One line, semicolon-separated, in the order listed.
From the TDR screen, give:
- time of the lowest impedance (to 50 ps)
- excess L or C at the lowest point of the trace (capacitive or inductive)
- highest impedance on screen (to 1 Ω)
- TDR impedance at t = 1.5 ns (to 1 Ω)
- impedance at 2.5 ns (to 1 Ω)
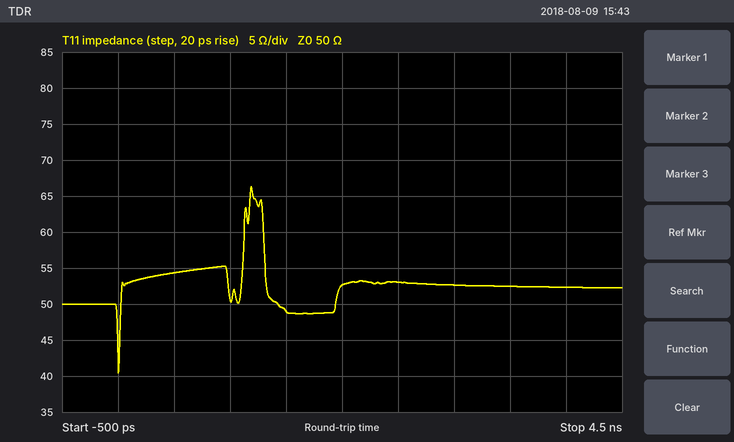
0 ps; capacitive; 66 Ω; 49 Ω; 53 Ω
